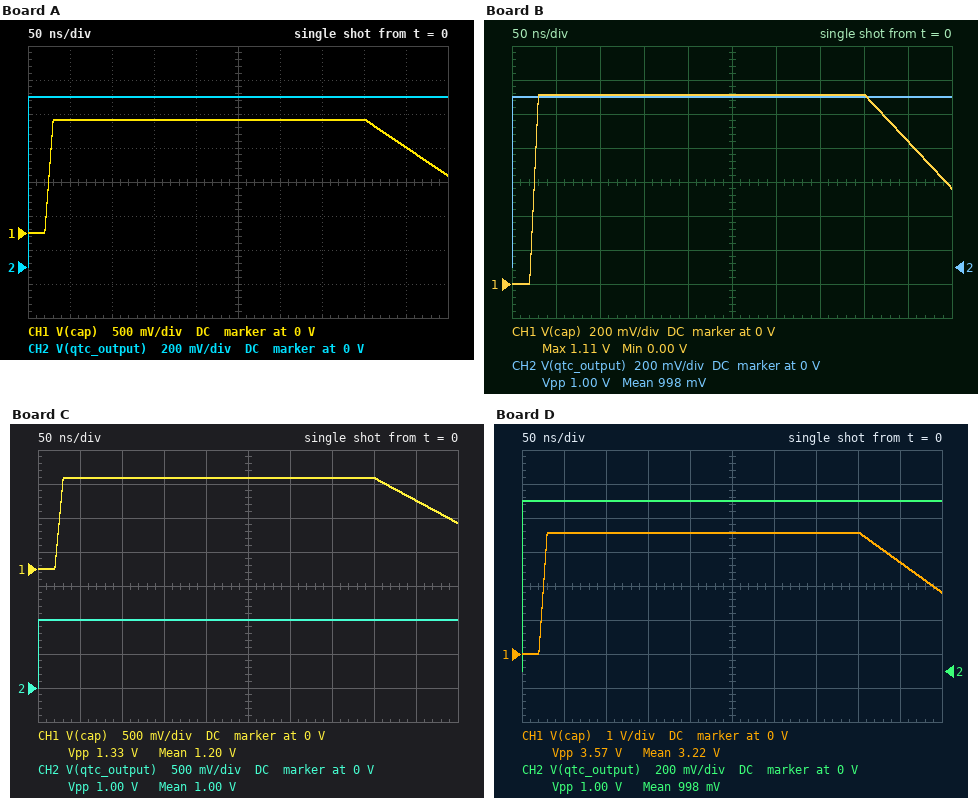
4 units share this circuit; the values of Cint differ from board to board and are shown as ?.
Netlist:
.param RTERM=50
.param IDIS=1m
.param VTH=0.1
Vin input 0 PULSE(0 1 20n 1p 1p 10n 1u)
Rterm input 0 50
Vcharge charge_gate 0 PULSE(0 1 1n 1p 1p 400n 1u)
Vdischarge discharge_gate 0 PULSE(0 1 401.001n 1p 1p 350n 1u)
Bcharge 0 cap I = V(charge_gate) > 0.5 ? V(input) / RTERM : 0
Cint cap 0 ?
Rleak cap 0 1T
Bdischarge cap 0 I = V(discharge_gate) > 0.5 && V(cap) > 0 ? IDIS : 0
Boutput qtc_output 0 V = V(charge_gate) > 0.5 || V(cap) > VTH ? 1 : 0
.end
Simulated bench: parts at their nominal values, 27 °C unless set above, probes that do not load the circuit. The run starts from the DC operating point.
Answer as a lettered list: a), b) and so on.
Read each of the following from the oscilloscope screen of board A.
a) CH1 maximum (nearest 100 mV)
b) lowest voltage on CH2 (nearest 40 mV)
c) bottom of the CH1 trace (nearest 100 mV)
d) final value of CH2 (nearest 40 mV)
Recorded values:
a) 1.7 V
b) 0 V
c) 0 V
d) 1.00 V
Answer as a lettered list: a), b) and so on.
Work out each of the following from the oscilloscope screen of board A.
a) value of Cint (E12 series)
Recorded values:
a) 120 pF
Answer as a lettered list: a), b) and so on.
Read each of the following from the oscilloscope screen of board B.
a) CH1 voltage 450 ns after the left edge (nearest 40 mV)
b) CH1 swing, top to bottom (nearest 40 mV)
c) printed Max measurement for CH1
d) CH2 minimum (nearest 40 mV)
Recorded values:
a) 840 mV
b) 1.12 V
c) 1.11 V
d) 0 V
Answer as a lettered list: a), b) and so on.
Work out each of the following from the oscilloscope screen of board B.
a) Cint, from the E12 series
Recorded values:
a) 180 pF
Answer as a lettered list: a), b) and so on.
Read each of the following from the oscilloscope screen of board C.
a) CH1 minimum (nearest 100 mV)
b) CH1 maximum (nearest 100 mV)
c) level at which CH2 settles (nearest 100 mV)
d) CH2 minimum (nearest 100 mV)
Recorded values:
a) 0 V
b) 1.3 V
c) 1.0 V
d) 0 V
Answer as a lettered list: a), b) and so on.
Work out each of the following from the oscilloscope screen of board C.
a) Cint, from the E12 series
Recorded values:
a) 150 pF
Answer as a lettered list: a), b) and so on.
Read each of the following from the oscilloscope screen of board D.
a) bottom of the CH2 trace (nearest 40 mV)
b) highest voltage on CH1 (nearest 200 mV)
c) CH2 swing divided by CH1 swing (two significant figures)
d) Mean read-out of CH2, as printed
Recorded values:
a) 0 V
b) 3.6 V
c) 0.28
d) 998 mV
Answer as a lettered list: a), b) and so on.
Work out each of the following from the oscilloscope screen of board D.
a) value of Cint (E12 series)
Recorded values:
a) 56 pF
